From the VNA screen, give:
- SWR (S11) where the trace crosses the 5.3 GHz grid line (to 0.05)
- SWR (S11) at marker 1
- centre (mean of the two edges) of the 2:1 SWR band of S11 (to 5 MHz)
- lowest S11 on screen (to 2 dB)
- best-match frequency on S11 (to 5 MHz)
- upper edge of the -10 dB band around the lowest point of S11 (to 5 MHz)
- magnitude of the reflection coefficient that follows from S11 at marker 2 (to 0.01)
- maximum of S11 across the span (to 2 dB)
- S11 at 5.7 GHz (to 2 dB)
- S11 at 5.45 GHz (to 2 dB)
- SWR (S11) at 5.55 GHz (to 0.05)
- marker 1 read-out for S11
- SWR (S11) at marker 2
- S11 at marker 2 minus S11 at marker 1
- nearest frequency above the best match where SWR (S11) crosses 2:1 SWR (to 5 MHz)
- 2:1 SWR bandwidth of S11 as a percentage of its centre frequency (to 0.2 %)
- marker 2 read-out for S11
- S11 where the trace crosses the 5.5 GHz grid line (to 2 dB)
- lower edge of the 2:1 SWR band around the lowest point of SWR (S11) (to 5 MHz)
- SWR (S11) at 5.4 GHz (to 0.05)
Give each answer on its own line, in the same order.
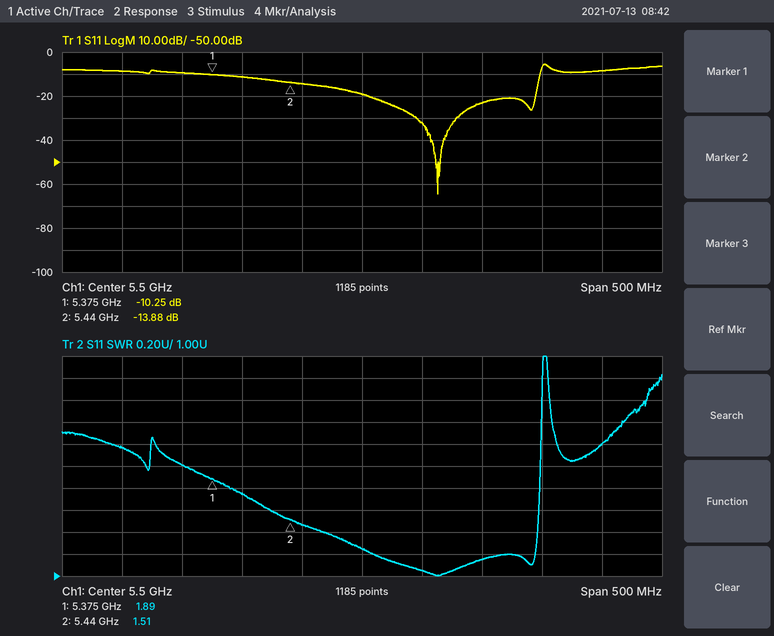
2.15
1.89
5.500 GHz
-64 dB
5.565 GHz
5.650 GHz
0.20
-6 dB
-8 dB
-14 dB
1.05
-10.25 dB
1.51
-3.63 dB
5.650 GHz
5.4 %
-13.88 dB
-20 dB
5.350 GHz
1.75
